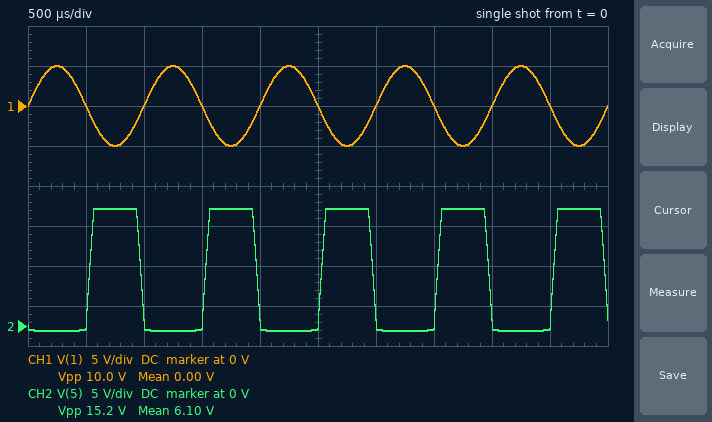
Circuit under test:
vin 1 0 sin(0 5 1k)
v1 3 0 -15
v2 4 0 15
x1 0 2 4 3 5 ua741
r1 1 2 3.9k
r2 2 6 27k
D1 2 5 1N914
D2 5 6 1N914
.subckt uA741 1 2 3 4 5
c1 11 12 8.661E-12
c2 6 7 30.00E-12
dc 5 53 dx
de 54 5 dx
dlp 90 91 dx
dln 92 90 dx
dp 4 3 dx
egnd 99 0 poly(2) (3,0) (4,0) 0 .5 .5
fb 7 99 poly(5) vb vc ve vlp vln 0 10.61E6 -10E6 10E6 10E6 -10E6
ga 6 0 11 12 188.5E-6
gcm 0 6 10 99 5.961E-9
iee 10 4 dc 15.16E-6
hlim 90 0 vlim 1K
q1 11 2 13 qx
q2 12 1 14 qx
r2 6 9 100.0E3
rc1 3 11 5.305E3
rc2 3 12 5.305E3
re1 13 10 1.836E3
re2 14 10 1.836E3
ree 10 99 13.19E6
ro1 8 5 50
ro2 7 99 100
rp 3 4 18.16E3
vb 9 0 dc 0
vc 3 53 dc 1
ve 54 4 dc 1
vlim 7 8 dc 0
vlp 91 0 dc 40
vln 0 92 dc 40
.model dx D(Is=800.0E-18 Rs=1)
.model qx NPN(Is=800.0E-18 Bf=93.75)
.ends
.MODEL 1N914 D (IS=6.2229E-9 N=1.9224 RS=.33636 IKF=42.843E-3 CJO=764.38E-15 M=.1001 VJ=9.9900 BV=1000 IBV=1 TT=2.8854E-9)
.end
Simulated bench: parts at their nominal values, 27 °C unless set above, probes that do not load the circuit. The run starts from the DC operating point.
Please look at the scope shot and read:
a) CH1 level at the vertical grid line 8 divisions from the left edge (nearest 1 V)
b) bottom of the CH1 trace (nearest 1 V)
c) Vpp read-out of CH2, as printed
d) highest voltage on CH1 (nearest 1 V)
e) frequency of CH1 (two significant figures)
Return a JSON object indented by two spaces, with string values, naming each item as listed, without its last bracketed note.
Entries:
{
  "CH1 level at the vertical grid line 8 divisions from the left edge": "0 V",
  "bottom of the CH1 trace": "-5 V",
  "Vpp read-out of CH2, as printed": "15.2 V",
  "highest voltage on CH1": "5 V",
  "frequency of CH1": "1.0 kHz"
}
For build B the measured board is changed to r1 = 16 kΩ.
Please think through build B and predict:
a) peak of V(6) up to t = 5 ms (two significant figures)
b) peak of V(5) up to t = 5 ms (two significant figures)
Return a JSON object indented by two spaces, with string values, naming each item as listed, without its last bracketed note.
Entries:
{
  "peak of V(6) up to t = 5 ms": "8.4 V",
  "peak of V(5) up to t = 5 ms": "9.0 V"
}
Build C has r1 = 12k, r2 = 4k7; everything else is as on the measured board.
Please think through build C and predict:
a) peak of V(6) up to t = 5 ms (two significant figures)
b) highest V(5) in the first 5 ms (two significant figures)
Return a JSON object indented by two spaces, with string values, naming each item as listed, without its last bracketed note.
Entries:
{
  "peak of V(6) up to t = 5 ms": "2.0 V",
  "highest V(5) in the first 5 ms": "2.5 V"
}
